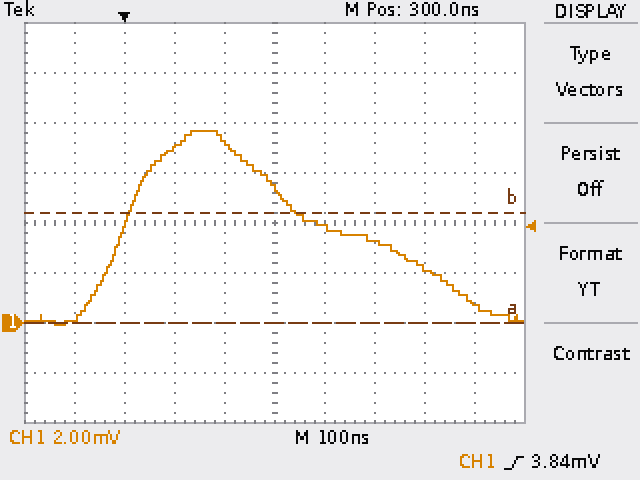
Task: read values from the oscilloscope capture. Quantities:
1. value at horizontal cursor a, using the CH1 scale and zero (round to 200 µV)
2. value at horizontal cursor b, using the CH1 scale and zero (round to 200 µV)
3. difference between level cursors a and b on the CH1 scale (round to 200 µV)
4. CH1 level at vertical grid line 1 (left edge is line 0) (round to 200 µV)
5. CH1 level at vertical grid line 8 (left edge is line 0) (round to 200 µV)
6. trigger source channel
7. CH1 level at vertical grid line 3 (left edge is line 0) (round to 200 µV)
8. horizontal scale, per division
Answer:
0.0 mV
4.4 mV
4.4 mV
200 µV
2.2 mV
CH1
7.0 mV
100 ns
